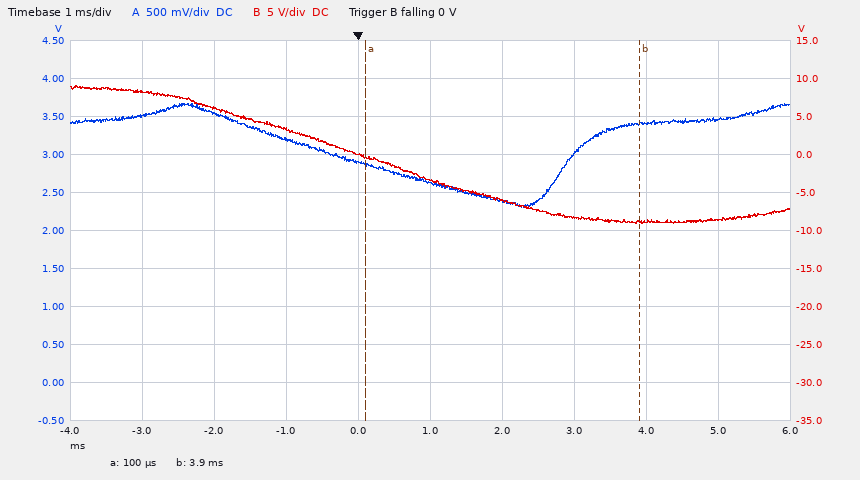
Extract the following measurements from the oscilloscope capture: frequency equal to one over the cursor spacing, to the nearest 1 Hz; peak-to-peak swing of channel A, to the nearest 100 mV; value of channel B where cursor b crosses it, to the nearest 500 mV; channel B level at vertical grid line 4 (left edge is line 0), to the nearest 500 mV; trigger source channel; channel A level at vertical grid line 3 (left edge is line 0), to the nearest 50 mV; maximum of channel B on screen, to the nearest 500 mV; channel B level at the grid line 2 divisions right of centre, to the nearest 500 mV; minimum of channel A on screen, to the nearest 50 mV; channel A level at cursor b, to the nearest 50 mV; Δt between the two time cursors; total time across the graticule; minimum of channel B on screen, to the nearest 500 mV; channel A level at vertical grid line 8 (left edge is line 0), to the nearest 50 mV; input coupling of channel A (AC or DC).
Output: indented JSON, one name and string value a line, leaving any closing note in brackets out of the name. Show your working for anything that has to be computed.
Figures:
{
  "frequency equal to one over the cursor spacing, to the nearest 1 Hz": "1 / 3.8 ms ≈ 263 Hz",
  "peak-to-peak swing of channel A, to the nearest 100 mV": "1.40 V",
  "value of channel B where cursor b crosses it, to the nearest 500 mV": "-9.0 V",
  "channel B level at vertical grid line 4 (left edge is line 0), to the nearest 500 mV": "0.0 V",
  "trigger source channel": "channel B",
  "channel A level at vertical grid line 3 (left edge is line 0), to the nearest 50 mV": "3.20 V",
  "maximum of channel B on screen, to the nearest 500 mV": "9.0 V",
  "channel B level at the grid line 2 divisions right of centre, to the nearest 500 mV": "-8.5 V",
  "minimum of channel A on screen, to the nearest 50 mV": "2.30 V",
  "channel A level at cursor b, to the nearest 50 mV": "3.40 V",
  "Δt between the two time cursors": "3.9 ms − (100 µs) = 3.8 ms",
  "total time across the graticule": "10 ms",
  "minimum of channel B on screen, to the nearest 500 mV": "-9.0 V",
  "channel A level at vertical grid line 8 (left edge is line 0), to the nearest 50 mV": "3.40 V",
  "input coupling of channel A": "DC"
}
